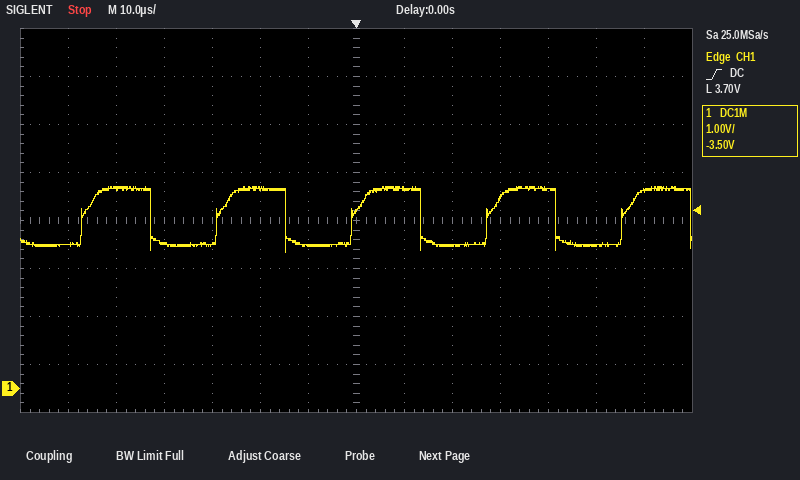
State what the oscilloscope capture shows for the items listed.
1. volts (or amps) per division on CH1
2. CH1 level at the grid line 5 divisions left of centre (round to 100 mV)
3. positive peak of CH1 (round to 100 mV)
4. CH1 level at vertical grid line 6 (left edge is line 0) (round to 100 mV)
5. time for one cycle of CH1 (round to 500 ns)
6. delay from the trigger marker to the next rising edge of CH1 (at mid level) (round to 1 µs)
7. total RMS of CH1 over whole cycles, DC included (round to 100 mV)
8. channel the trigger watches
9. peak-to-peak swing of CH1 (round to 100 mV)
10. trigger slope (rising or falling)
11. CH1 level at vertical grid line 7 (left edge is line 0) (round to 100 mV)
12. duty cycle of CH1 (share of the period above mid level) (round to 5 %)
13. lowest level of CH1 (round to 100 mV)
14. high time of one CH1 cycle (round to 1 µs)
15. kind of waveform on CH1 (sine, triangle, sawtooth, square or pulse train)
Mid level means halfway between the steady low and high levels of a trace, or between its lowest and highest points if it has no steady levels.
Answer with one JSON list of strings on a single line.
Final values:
["1 V", "4.2 V", "4.2 V", "3.0 V", "28.0 µs", "27 µs", "3.6 V", "CH1", "1.4 V", "rising", "3.7 V", "50 %", "2.8 V", "14 µs", "square"]
